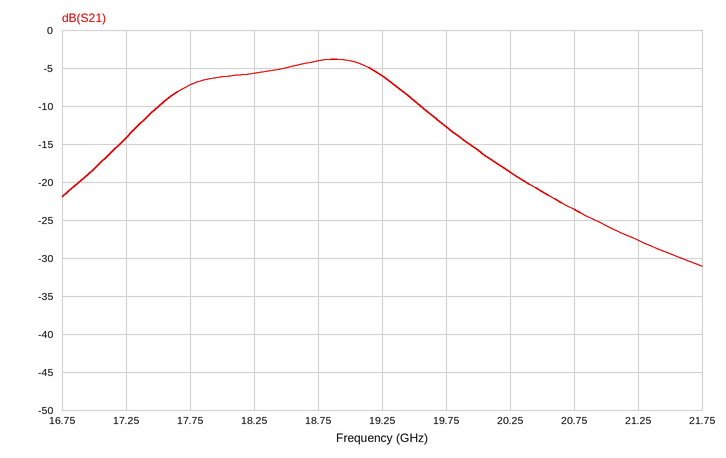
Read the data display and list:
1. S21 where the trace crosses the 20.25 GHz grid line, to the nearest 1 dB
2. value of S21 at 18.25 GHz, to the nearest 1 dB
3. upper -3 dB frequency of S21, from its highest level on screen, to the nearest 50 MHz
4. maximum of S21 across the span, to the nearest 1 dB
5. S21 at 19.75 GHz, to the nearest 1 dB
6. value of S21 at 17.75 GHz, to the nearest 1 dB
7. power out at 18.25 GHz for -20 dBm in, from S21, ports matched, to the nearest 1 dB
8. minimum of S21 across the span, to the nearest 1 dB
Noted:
-19 dB
-6 dB
19.30 GHz
-4 dB
-13 dB
-7 dB
-26 dBm
-31 dB
